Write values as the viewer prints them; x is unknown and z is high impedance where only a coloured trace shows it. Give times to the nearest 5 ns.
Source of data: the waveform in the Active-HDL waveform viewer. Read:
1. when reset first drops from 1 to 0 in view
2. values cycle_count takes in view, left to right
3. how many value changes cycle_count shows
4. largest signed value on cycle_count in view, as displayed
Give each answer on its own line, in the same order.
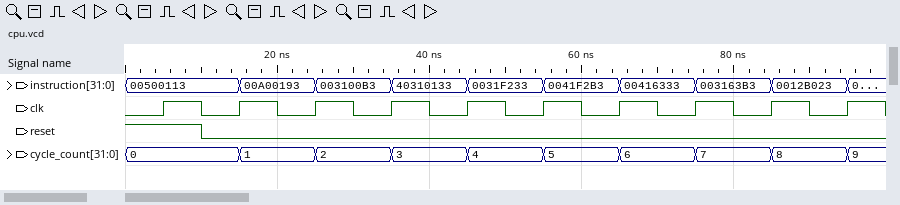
10 ns
0, 1, 2, 3, 4, 5, 6, 7, 8, 9
9
9
